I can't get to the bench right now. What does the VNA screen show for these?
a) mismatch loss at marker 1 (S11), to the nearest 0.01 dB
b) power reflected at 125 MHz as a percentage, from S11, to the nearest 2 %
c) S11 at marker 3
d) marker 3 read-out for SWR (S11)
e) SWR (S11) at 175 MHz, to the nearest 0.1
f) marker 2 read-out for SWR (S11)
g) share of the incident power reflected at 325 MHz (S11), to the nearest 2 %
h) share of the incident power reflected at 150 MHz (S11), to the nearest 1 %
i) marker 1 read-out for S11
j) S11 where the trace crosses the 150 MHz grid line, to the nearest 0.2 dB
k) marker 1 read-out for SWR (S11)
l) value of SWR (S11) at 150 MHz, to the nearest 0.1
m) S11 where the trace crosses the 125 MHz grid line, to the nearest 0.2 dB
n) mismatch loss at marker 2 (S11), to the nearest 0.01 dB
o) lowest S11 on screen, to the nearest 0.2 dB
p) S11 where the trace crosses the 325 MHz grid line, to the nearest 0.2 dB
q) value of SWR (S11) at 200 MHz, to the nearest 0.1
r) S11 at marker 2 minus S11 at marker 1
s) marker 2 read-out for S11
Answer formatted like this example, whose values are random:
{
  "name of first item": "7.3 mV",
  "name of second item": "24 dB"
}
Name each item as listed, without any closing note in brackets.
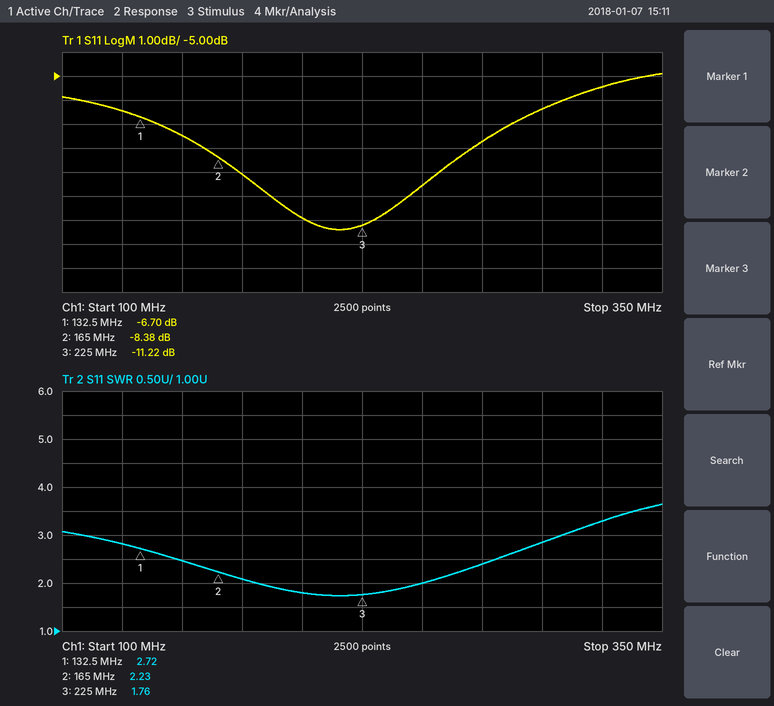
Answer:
{
  "mismatch loss at marker 1 (S11), to the nearest 0.01 dB": "1.04 dB",
  "power reflected at 125 MHz as a percentage, from S11, to the nearest 2 %": "22 %",
  "S11 at marker 3": "-11.22 dB",
  "marker 3 read-out for SWR": "1.76",
  "SWR (S11) at 175 MHz, to the nearest 0.1": "2.1",
  "marker 2 read-out for SWR": "2.23",
  "share of the incident power reflected at 325 MHz (S11), to the nearest 2 %": "28 %",
  "share of the incident power reflected at 150 MHz (S11), to the nearest 1 %": "18 %",
  "marker 1 read-out for S11": "-6.70 dB",
  "S11 where the trace crosses the 150 MHz grid line, to the nearest 0.2 dB": "-7.4 dB",
  "marker 1 read-out for SWR": "2.72",
  "value of SWR (S11) at 150 MHz, to the nearest 0.1": "2.5",
  "S11 where the trace crosses the 125 MHz grid line, to the nearest 0.2 dB": "-6.4 dB",
  "mismatch loss at marker 2 (S11), to the nearest 0.01 dB": "0.68 dB",
  "lowest S11 on screen, to the nearest 0.2 dB": "-11.4 dB",
  "S11 where the trace crosses the 325 MHz grid line, to the nearest 0.2 dB": "-5.4 dB",
  "value of SWR (S11) at 200 MHz, to the nearest 0.1": "1.8",
  "S11 at marker 2 minus S11 at marker 1": "-1.68 dB",
  "marker 2 read-out for S11": "-8.38 dB"
}
